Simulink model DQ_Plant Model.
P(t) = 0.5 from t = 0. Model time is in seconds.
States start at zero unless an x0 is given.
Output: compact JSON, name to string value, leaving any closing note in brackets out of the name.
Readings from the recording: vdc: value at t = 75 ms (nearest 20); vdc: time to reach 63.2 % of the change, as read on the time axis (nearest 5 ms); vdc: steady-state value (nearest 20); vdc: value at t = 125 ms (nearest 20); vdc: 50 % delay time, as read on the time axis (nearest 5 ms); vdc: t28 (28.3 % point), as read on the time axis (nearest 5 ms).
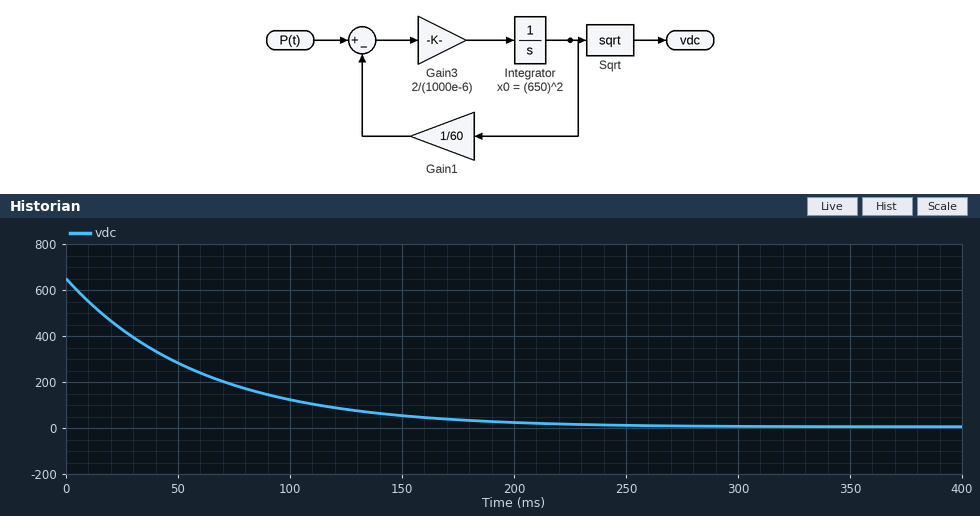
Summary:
{"vdc: value at t = 75 ms": "180", "vdc: time to reach 63.2 % of the change, as read on the time axis": "60 ms", "vdc: steady-state value": "0", "vdc: value at t = 125 ms": "80", "vdc: 50 % delay time, as read on the time axis": "40 ms", "vdc: t28 (28.3 % point), as read on the time axis": "20 ms"}
